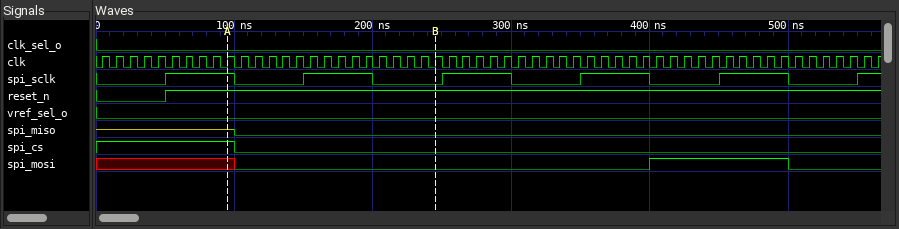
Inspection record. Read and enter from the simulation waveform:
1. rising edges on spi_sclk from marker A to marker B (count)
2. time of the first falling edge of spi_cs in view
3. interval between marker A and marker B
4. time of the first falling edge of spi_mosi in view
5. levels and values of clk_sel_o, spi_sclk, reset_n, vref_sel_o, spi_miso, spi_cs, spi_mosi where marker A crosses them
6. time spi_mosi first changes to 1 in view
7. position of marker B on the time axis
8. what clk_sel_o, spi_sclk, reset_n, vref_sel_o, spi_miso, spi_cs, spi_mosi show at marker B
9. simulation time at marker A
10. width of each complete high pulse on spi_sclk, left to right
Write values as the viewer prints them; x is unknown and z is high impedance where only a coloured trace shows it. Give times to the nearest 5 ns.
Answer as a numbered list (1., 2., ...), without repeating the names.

1. 1
2. 100 ns
3. 150 ns
4. 500 ns
5. clk_sel_o=0, spi_sclk=1, reset_n=1, vref_sel_o=0, spi_miso=z, spi_cs=1, spi_mosi=x
6. 400 ns
7. 245 ns
8. clk_sel_o=0, spi_sclk=0, reset_n=1, vref_sel_o=0, spi_miso=0, spi_cs=0, spi_mosi=0
9. 95 ns
10. 50 ns, 50 ns, 50 ns, 50 ns, 50 ns
